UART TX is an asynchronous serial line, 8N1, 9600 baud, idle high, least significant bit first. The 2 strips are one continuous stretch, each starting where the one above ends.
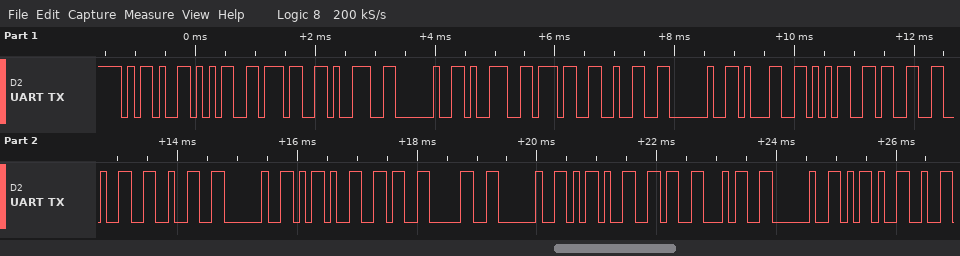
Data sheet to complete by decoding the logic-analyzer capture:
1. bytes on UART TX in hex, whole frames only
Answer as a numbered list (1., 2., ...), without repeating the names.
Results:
1. 2D 35 37 39 20 39 37 32 20 31 35 33 32 32 20 2D 36 30 20 2D 36 34 20 2D
